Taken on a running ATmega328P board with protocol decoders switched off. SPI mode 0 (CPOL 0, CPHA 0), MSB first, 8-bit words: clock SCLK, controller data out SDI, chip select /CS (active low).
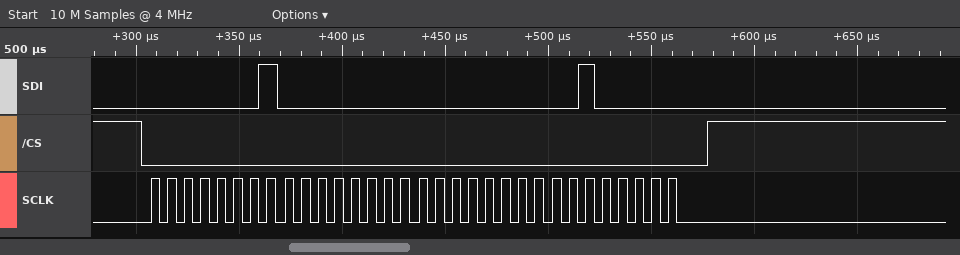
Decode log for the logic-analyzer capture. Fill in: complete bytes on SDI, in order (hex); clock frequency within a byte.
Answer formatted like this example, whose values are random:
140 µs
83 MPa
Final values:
01 00 00 20
125 kHz
